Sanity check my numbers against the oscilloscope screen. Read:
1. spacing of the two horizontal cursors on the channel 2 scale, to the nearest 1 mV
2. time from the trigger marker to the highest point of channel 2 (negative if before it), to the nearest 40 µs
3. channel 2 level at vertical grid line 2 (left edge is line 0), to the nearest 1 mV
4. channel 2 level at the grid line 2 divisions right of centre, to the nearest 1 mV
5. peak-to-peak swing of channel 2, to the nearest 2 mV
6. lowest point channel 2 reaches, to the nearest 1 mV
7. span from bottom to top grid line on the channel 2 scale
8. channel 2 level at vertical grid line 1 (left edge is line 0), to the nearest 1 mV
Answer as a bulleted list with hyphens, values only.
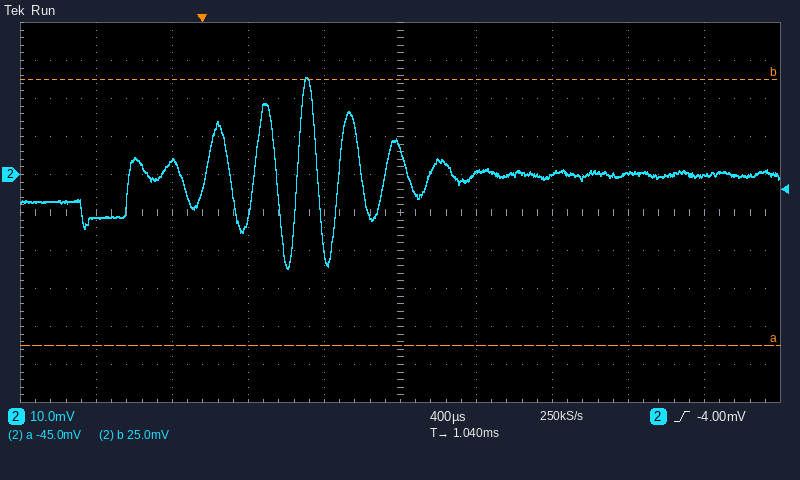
- 70 mV
- +560 µs
- 3 mV
- 0 mV
- 50 mV
- -25 mV
- 100 mV
- -11 mV
